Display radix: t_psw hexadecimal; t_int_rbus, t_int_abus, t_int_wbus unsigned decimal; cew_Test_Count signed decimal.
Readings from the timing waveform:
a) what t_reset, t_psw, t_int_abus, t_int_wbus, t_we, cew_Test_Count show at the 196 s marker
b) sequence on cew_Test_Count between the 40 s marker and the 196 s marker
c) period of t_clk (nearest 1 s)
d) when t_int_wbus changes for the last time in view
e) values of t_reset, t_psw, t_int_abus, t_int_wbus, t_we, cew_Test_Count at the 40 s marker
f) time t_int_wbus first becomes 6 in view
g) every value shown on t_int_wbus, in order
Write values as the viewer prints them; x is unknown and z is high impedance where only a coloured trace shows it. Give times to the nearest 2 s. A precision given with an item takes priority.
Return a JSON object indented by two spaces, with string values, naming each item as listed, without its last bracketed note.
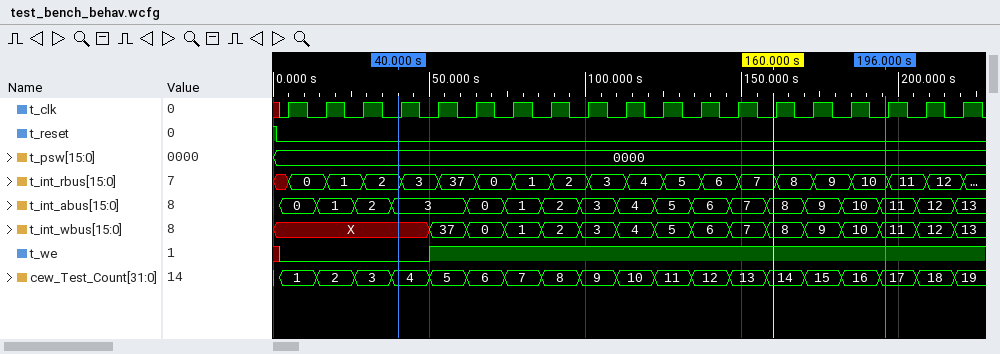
{
  "what t_reset, t_psw, t_int_abus, t_int_wbus, t_we, cew_Test_Count show at the 196 s marker": "t_reset=0, t_psw=0000, t_int_abus=11, t_int_wbus=11, t_we=1, cew_Test_Count=17",
  "sequence on cew_Test_Count between the 40 s marker and the 196 s marker": "4, 5, 6, 7, 8, 9, 10, 11, 12, 13, 14, 15, 16, 17",
  "period of t_clk": "12 s",
  "when t_int_wbus changes for the last time in view": "218 s",
  "values of t_reset, t_psw, t_int_abus, t_int_wbus, t_we, cew_Test_Count at the 40 s marker": "t_reset=0, t_psw=0000, t_int_abus=3, t_int_wbus=X, t_we=0, cew_Test_Count=4",
  "time t_int_wbus first becomes 6 in view": "134 s",
  "every value shown on t_int_wbus, in order": "X, 37, 0, 1, 2, 3, 4, 5, 6, 7, 8, 9, 10, 11, 12, 13"
}
